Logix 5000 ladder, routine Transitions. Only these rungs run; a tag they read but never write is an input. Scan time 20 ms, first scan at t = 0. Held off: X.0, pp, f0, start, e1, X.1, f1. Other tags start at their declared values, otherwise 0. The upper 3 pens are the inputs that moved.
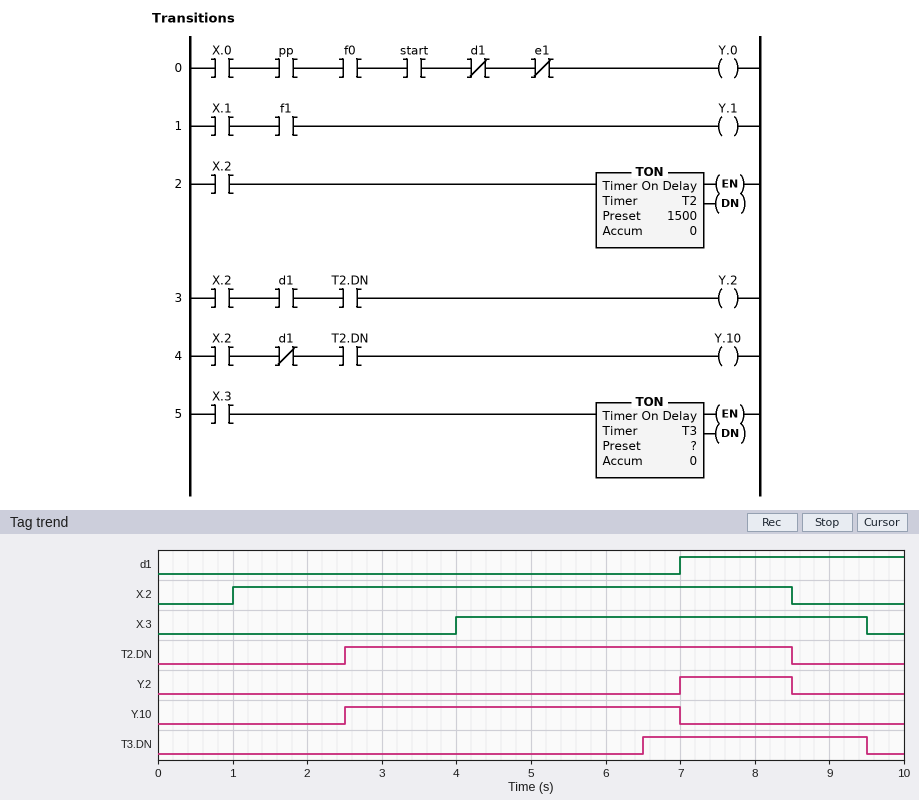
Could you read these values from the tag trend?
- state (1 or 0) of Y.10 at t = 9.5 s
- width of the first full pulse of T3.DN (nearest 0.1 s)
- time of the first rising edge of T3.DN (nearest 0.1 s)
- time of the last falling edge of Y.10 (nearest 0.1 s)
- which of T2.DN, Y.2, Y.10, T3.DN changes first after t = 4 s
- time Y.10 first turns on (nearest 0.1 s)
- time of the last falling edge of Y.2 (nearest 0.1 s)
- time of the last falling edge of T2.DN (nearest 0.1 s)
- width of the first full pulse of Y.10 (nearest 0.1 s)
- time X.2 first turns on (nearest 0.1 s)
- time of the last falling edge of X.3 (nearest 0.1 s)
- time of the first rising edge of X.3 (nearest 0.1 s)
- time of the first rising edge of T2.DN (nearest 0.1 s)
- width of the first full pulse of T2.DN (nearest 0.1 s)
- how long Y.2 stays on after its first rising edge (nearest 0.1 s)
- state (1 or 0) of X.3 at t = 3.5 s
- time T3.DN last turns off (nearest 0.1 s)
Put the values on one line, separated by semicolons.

0; 3.0 s; 6.5 s; 7.0 s; T3.DN; 2.5 s; 8.5 s; 8.5 s; 4.5 s; 1.0 s; 9.5 s; 4.0 s; 2.5 s; 6.0 s; 1.5 s; 0; 9.5 s
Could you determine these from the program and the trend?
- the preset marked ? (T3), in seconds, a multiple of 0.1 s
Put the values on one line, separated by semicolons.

2.5 s
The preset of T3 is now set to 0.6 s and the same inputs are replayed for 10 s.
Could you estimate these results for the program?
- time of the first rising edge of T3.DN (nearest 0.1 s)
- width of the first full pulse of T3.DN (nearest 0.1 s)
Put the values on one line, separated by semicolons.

4.6 s; 4.9 s
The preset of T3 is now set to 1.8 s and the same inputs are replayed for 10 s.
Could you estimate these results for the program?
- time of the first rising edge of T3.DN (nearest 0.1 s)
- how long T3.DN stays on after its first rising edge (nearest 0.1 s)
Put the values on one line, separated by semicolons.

5.8 s; 3.7 s
